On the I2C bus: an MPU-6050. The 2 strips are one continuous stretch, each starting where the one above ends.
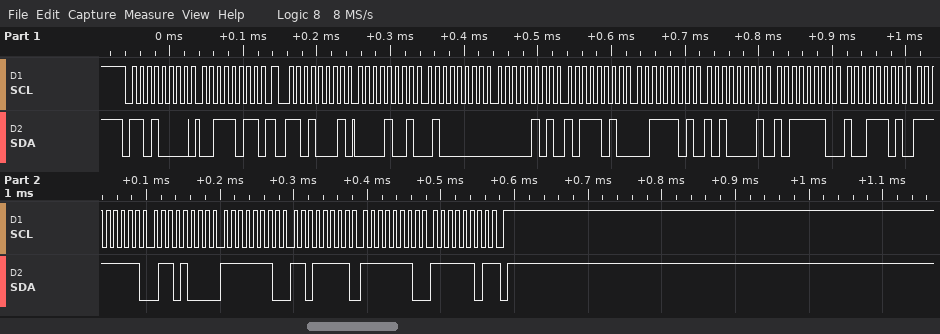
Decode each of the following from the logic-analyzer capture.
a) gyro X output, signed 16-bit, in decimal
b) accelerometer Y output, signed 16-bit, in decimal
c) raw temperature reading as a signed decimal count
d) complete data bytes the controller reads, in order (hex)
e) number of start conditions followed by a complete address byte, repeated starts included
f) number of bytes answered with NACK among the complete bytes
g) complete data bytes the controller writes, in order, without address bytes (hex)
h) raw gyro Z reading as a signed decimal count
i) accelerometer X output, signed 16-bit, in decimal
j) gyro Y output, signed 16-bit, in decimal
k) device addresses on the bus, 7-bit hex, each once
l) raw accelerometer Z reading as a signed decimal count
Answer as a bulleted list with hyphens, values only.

- -152
- 1466
- -16739
- 09 40 05 BA 3D A1 BE 9D FF 68 FE DF FE FD
- 2
- 1
- 3B
- -259
- 2368
- -289
- 0x68
- 15777
